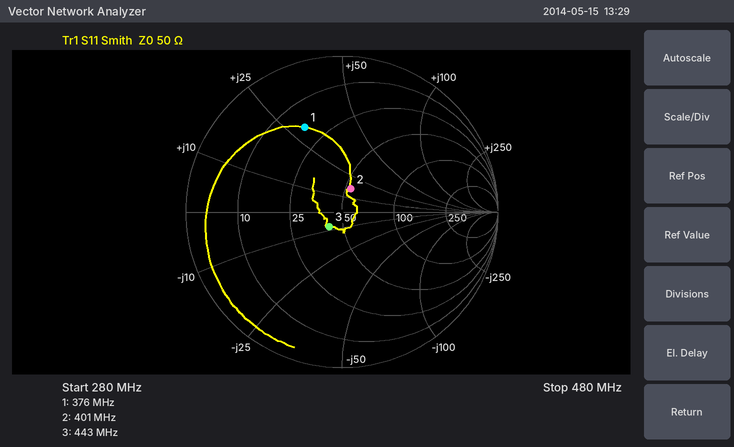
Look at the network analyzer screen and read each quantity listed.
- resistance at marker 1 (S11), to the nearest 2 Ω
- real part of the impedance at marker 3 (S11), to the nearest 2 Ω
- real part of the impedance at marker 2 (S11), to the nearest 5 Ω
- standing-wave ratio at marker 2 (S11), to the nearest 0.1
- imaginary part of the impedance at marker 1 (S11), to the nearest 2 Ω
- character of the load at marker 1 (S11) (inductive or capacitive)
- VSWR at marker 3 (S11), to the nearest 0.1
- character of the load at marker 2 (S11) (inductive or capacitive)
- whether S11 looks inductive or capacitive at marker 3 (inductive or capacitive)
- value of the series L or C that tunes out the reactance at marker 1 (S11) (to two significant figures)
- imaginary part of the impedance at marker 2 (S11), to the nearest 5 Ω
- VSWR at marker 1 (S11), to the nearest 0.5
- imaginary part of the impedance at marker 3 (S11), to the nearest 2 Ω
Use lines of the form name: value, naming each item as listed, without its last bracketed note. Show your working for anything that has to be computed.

resistance at marker 1 (S11), to the nearest 2 Ω: 18 Ω
real part of the impedance at marker 3 (S11), to the nearest 2 Ω: 42 Ω
real part of the impedance at marker 2 (S11), to the nearest 5 Ω: 55 Ω
standing-wave ratio at marker 2 (S11), to the nearest 0.1: 1.4
imaginary part of the impedance at marker 1 (S11), to the nearest 2 Ω: +30 Ω
character of the load at marker 1 (S11): inductive
VSWR at marker 3 (S11), to the nearest 0.1: 1.3
character of the load at marker 2 (S11): inductive
whether S11 looks inductive or capacitive at marker 3: capacitive
value of the series L or C that tunes out the reactance at marker 1 (S11): C = 1/(2π × 376 MHz × 30 Ω) ≈ 14 pF
imaginary part of the impedance at marker 2 (S11), to the nearest 5 Ω: +15 Ω
VSWR at marker 1 (S11), to the nearest 0.5: 4.0
imaginary part of the impedance at marker 3 (S11), to the nearest 2 Ω: -8 Ω
